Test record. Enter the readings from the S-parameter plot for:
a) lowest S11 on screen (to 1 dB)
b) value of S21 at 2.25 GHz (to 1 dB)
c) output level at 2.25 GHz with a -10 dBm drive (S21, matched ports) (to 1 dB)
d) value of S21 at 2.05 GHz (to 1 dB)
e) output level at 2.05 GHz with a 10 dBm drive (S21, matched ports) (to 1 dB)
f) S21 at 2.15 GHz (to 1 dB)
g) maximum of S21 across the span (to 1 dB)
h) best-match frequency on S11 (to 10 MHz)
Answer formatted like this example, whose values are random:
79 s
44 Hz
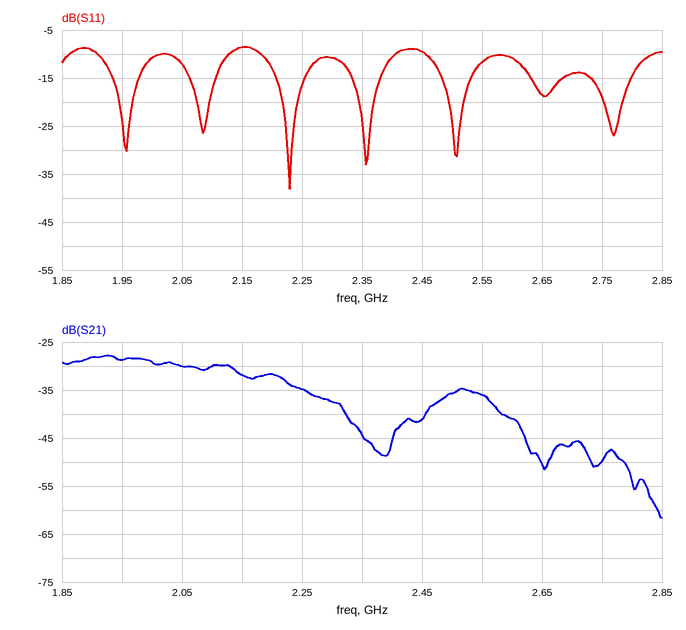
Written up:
-38 dB
-35 dB
-45 dBm
-30 dB
-20 dBm
-32 dB
-28 dB
2.23 GHz
